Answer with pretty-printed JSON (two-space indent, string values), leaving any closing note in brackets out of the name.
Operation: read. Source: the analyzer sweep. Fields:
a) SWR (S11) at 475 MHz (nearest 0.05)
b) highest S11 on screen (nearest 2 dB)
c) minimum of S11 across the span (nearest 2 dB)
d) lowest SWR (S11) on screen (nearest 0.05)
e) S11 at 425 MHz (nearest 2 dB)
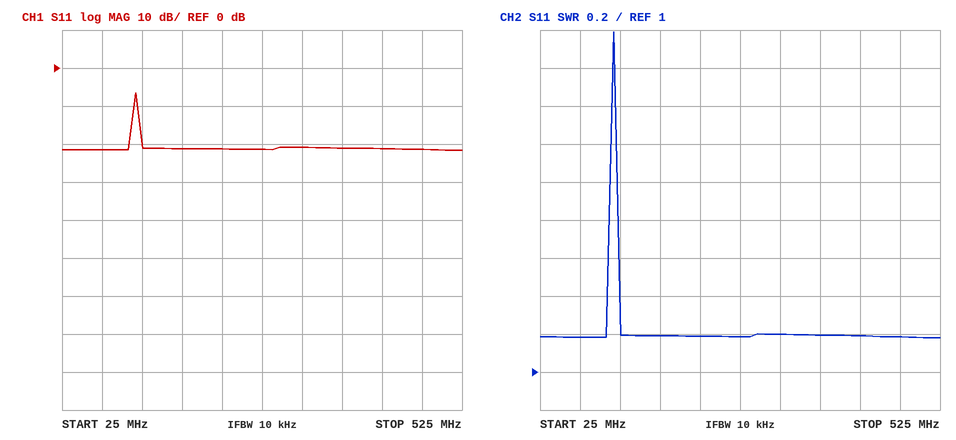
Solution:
{
  "SWR (S11) at 475 MHz": "1.20",
  "highest S11 on screen": "-6 dB",
  "minimum of S11 across the span": "-22 dB",
  "lowest SWR (S11) on screen": "1.20",
  "S11 at 425 MHz": "-22 dB"
}
